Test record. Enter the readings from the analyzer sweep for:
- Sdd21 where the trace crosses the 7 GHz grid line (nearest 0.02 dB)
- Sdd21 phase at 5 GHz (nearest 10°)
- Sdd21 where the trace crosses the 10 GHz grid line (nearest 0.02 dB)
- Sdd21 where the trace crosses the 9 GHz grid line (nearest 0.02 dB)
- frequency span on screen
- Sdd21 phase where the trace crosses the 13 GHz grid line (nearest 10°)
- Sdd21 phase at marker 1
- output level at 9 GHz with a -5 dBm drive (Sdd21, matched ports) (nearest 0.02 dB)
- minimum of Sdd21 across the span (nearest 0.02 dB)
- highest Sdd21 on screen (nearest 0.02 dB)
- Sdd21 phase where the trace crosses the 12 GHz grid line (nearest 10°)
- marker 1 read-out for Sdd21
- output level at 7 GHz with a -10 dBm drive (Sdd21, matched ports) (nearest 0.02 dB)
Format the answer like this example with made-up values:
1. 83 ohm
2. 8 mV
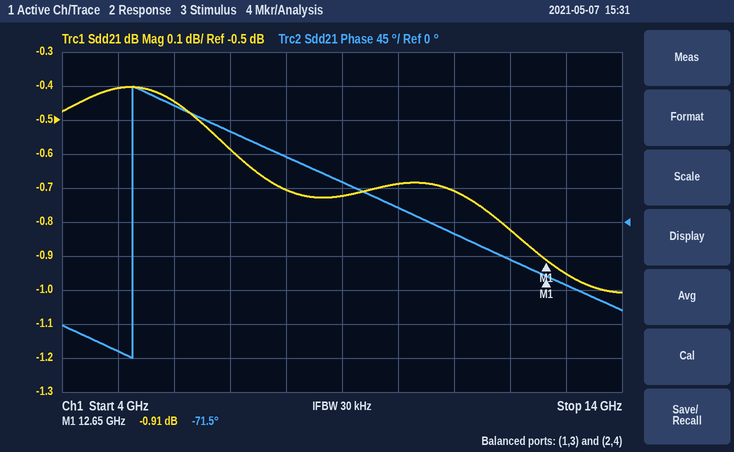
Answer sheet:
1. -0.58 dB
2. -170°
3. -0.68 dB
4. -0.72 dB
5. 10 GHz
6. -80°
7. -71.5°
8. -5.72 dBm
9. -1.00 dB
10. -0.40 dB
11. -50°
12. -0.91 dB
13. -10.58 dBm
